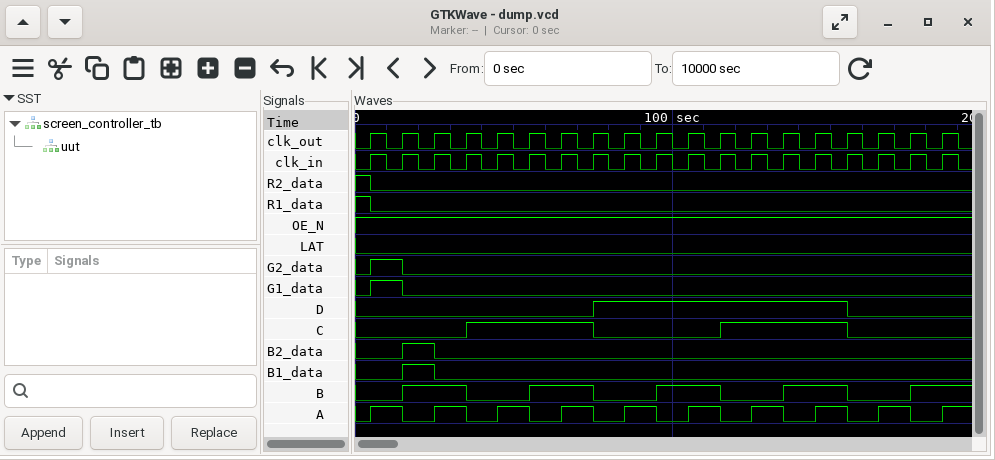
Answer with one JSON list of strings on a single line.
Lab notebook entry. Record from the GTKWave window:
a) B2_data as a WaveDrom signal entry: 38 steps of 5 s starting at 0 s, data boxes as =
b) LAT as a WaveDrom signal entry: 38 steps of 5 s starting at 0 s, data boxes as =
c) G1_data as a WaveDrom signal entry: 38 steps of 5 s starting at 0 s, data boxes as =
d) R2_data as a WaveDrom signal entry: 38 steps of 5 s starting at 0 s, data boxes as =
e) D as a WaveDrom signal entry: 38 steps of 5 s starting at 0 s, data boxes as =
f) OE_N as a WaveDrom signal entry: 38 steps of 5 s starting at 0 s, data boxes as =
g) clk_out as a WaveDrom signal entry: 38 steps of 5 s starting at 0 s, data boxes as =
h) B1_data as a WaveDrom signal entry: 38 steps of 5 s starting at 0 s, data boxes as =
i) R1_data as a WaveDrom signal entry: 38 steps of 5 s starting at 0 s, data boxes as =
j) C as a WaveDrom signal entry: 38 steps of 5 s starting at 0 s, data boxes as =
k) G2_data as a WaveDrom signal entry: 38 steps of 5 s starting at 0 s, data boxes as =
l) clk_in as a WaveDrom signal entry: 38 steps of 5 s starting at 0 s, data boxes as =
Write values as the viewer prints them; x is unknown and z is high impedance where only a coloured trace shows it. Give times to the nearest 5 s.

["{name: 'B2_data', wave: '0..1.0................................'}", "{name: 'LAT', wave: '0.....................................'}", "{name: 'G1_data', wave: '01.0..................................'}", "{name: 'R2_data', wave: '10....................................'}", "{name: 'D', wave: '0..............1...............0......'}", "{name: 'OE_N', wave: '1.....................................'}", "{name: 'clk_out', wave: '01010101010101010101010101010101010101'}", "{name: 'B1_data', wave: '0..1.0................................'}", "{name: 'R1_data', wave: '10....................................'}", "{name: 'C', wave: '0......1.......0.......1.......0......'}", "{name: 'G2_data', wave: '01.0..................................'}", "{name: 'clk_in', wave: '01010101010101010101010101010101010101'}"]
